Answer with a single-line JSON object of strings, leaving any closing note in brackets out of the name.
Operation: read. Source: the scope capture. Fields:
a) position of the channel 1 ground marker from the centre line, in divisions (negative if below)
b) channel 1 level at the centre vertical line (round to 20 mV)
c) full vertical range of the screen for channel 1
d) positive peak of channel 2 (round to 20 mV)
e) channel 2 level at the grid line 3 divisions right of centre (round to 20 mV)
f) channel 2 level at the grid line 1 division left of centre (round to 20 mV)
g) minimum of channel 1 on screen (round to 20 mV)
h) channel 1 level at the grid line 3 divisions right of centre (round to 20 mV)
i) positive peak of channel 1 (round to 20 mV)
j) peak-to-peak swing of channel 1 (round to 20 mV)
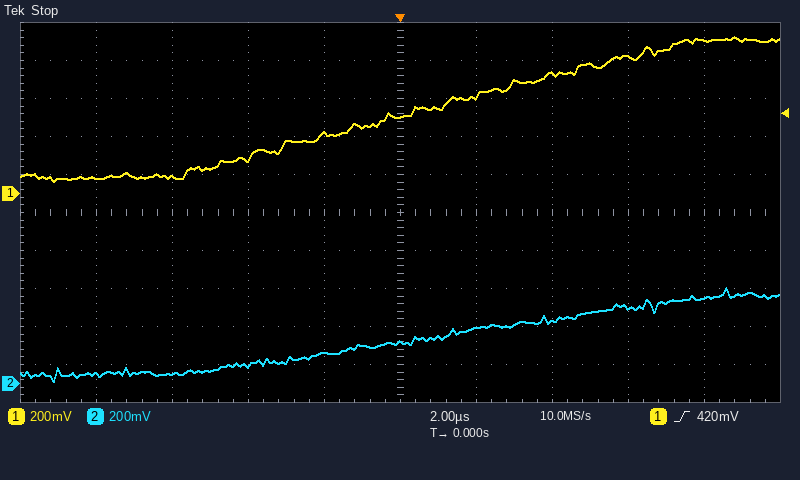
{"position of the channel 1 ground marker from the centre line, in divisions": "+0.5 div", "channel 1 level at the centre vertical line": "400 mV", "full vertical range of the screen for channel 1": "2 V", "positive peak of channel 2": "500 mV", "channel 2 level at the grid line 3 divisions right of centre": "400 mV", "channel 2 level at the grid line 1 division left of centre": "160 mV", "minimum of channel 1 on screen": "60 mV", "channel 1 level at the grid line 3 divisions right of centre": "720 mV", "positive peak of channel 1": "820 mV", "peak-to-peak swing of channel 1": "760 mV"}
